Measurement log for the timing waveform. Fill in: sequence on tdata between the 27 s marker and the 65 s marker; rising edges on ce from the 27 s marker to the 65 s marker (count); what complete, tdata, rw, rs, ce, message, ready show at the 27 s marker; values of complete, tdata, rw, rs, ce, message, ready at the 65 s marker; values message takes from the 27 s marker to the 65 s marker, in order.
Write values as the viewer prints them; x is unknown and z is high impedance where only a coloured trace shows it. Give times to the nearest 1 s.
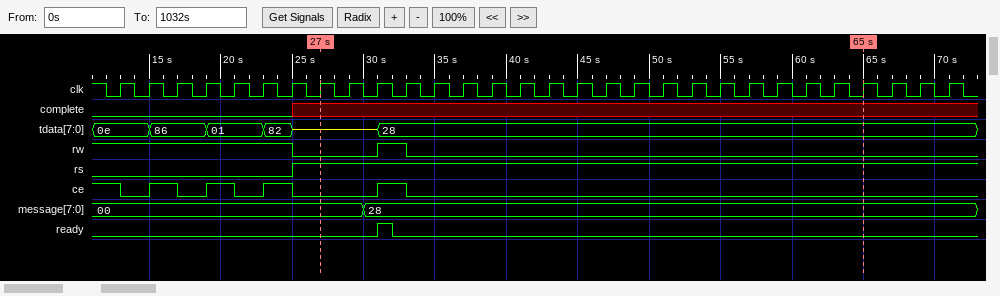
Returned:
z, 28
1
complete=x, tdata=z, rw=0, rs=1, ce=0, message=00, ready=0
complete=x, tdata=28, rw=0, rs=1, ce=0, message=28, ready=0
00, 28
